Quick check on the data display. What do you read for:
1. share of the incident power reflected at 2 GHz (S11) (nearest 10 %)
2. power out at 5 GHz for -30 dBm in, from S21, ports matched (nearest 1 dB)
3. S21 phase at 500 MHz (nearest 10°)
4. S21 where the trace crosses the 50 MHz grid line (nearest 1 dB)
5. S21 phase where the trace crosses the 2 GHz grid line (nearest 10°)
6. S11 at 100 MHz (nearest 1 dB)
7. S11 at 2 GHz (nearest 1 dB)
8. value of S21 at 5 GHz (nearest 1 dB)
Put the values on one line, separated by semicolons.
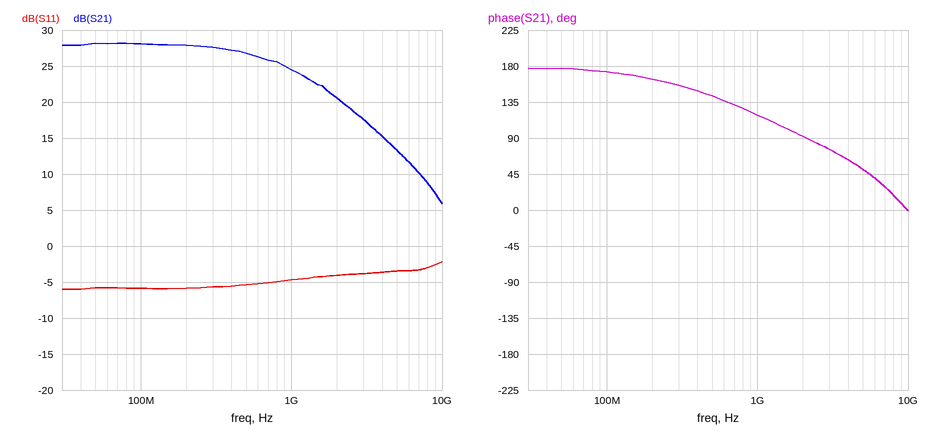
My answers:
40 %; -17 dBm; 140°; 28 dB; 90°; -6 dB; -4 dB; 13 dB
